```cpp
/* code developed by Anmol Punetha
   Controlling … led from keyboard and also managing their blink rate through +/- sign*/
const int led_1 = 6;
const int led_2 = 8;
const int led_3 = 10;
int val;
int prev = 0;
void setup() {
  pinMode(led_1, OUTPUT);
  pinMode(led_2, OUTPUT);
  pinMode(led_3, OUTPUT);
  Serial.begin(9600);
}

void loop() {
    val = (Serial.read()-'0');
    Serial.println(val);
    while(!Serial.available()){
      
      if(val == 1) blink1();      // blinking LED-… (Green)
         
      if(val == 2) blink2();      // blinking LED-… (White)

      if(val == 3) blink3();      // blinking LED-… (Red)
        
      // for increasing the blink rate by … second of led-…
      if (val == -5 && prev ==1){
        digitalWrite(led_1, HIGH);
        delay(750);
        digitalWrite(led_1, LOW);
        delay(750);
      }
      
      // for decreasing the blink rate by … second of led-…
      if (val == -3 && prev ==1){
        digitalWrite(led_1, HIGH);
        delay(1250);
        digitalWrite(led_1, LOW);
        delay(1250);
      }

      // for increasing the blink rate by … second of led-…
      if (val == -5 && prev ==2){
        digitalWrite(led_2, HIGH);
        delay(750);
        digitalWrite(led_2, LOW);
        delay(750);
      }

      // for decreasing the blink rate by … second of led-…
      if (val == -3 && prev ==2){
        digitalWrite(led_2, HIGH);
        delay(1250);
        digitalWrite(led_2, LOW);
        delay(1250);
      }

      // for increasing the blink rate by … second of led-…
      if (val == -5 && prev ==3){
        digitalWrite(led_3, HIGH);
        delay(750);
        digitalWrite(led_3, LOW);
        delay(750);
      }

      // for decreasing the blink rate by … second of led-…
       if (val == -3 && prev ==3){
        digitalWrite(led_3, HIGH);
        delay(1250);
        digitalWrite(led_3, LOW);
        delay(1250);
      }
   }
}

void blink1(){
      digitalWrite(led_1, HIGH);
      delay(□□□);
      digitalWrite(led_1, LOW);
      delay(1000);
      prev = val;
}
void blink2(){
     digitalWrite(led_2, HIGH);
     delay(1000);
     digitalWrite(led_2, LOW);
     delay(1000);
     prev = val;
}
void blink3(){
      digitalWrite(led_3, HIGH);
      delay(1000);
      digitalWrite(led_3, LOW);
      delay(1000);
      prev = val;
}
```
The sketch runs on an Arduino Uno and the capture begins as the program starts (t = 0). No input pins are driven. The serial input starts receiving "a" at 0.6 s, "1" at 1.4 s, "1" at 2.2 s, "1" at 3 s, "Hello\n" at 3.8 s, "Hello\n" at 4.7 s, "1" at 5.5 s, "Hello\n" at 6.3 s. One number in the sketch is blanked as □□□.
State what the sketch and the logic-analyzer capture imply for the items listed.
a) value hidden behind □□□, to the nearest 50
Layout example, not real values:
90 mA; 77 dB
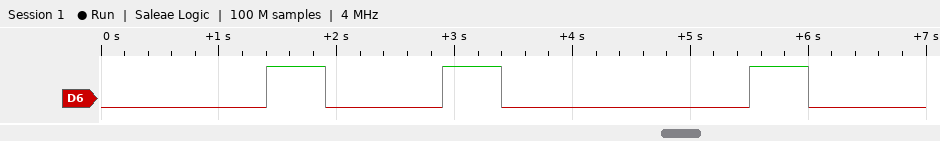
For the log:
500
